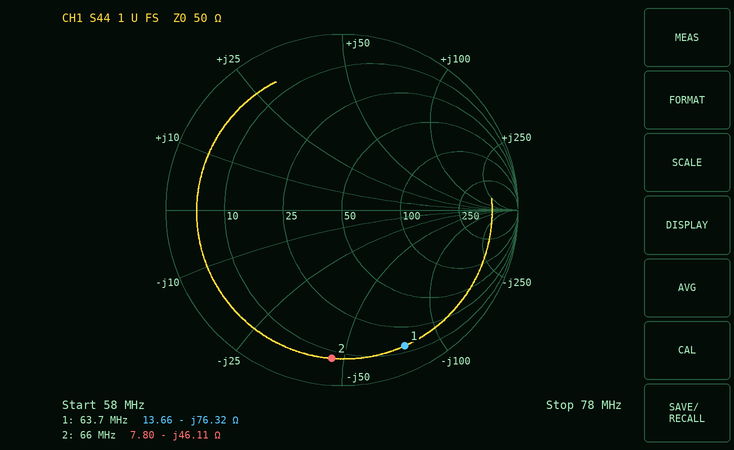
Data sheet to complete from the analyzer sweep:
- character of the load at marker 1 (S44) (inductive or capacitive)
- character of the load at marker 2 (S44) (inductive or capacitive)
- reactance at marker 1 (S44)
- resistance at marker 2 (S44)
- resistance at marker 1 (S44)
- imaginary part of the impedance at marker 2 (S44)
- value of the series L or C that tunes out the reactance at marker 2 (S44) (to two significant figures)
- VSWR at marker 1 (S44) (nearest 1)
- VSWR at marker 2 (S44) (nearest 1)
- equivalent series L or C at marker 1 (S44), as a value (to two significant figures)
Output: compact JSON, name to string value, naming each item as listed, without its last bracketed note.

{"character of the load at marker 1 (S44)": "capacitive", "character of the load at marker 2 (S44)": "capacitive", "reactance at marker 1": "-76.32 Ω", "resistance at marker 2": "7.80 Ω", "resistance at marker 1": "13.66 Ω", "imaginary part of the impedance at marker 2": "-46.11 Ω", "value of the series L or C that tunes out the reactance at marker 2 (S44)": "110 nH", "VSWR at marker 1 (S44)": "12", "VSWR at marker 2 (S44)": "12", "equivalent series L or C at marker 1 (S44), as a value": "33 pF"}
